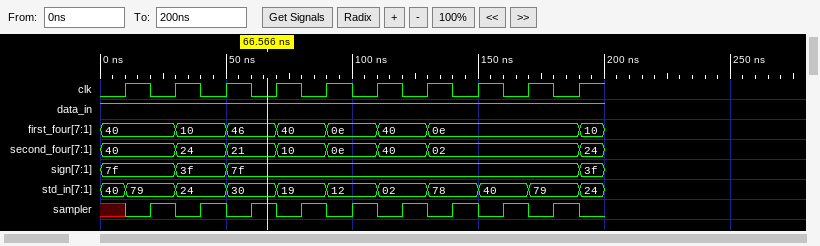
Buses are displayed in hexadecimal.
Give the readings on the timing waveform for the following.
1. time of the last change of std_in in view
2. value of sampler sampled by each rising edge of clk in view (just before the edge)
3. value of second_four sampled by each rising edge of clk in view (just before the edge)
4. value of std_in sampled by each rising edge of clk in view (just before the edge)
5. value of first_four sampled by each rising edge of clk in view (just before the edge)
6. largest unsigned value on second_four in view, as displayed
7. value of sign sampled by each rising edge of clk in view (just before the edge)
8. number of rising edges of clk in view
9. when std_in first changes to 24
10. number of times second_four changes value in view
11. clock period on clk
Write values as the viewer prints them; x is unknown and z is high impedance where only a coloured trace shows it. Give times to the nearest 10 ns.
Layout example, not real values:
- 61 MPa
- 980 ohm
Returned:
- 190 ns
- x 1 1 1 1 1 1 1 1 1
- 40, 40, 24, 21, 10, 0e, 40, 02, 02, 02
- 40, 79, 24, 30, 19, 12, 02, 78, 40, 79
- 40, 40, 10, 46, 40, 0e, 40, 0e, 0e, 0e
- 40
- 7f, 7f, 3f, 7f, 7f, 7f, 7f, 7f, 7f, 7f
- 10
- 30 ns
- 7
- 20 ns
